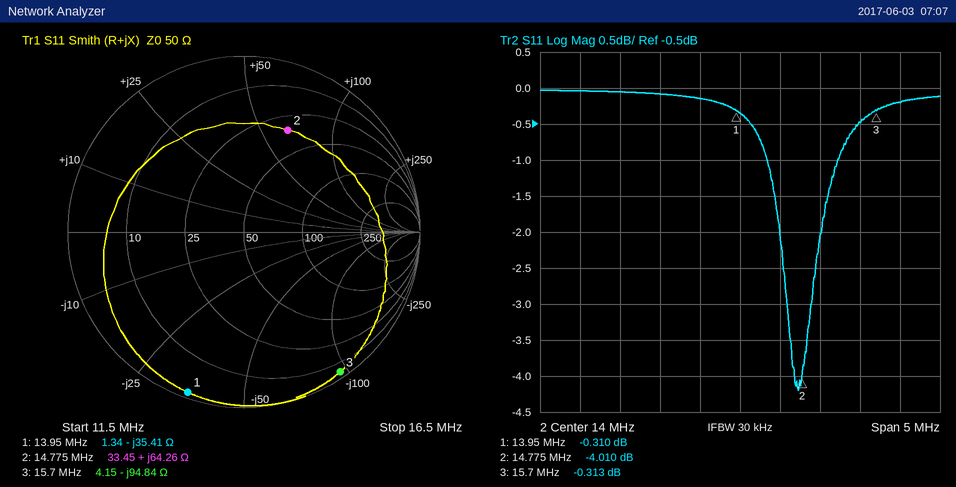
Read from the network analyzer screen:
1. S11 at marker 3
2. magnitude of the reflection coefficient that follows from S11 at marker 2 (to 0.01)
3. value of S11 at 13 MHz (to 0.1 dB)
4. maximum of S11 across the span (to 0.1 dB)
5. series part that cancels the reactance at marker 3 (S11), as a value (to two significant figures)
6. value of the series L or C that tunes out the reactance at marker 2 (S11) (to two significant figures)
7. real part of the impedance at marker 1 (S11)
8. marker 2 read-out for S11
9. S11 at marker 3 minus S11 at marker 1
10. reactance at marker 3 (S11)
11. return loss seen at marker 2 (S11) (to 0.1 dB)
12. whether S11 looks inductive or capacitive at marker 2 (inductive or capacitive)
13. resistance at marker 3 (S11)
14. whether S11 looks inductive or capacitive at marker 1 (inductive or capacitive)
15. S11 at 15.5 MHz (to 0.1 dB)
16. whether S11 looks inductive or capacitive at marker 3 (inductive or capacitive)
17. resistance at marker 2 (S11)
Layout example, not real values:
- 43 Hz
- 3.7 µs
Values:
- -0.313 dB
- 0.63
- -0.1 dB
- 0.0 dB
- 960 nH
- 170 pF
- 1.34 Ω
- -4.010 dB
- -0.003 dB
- -94.84 Ω
- 4.0 dB
- inductive
- 4.15 Ω
- capacitive
- -0.5 dB
- capacitive
- 33.45 Ω
